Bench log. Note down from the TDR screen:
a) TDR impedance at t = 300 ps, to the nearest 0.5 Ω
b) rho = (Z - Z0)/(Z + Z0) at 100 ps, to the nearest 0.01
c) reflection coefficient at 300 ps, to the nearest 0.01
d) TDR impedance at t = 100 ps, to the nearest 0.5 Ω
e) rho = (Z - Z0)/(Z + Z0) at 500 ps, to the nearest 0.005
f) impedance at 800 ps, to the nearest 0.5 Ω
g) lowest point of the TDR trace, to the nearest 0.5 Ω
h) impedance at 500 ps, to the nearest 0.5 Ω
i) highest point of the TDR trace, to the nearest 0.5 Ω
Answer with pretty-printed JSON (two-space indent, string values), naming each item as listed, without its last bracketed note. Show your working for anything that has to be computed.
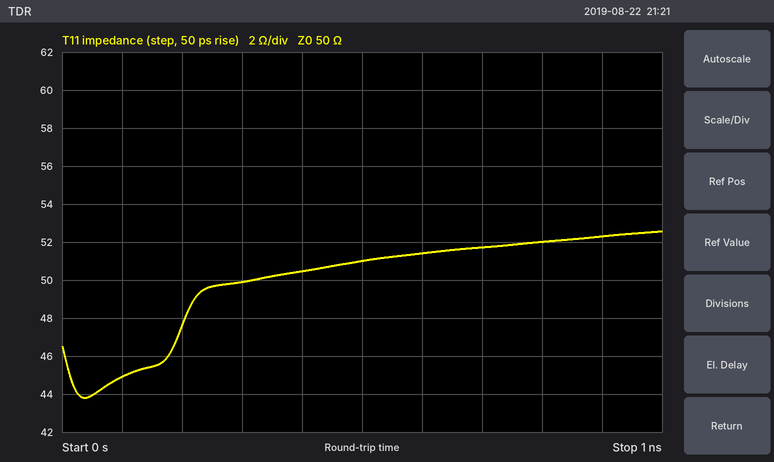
{
  "TDR impedance at t = 300 ps, to the nearest 0.5 Ω": "50.0 Ω",
  "rho = (Z - Z0)/(Z + Z0) at 100 ps, to the nearest 0.01": "(45 − 50)/(45 + 50) ≈ -0.05",
  "reflection coefficient at 300 ps, to the nearest 0.01": "(50 − 50)/(50 + 50) ≈ 0.00",
  "TDR impedance at t = 100 ps, to the nearest 0.5 Ω": "45.0 Ω",
  "rho = (Z - Z0)/(Z + Z0) at 500 ps, to the nearest 0.005": "(51 − 50)/(51 + 50) ≈ +0.010",
  "impedance at 800 ps, to the nearest 0.5 Ω": "52.0 Ω",
  "lowest point of the TDR trace, to the nearest 0.5 Ω": "44.0 Ω",
  "impedance at 500 ps, to the nearest 0.5 Ω": "51.0 Ω",
  "highest point of the TDR trace, to the nearest 0.5 Ω": "52.5 Ω"
}
